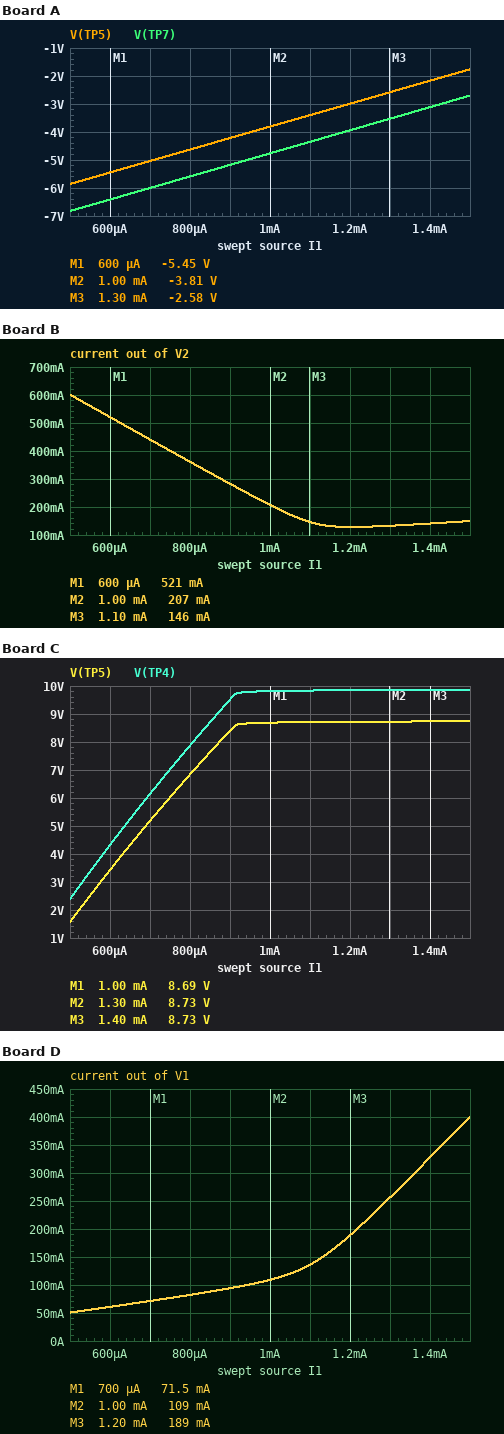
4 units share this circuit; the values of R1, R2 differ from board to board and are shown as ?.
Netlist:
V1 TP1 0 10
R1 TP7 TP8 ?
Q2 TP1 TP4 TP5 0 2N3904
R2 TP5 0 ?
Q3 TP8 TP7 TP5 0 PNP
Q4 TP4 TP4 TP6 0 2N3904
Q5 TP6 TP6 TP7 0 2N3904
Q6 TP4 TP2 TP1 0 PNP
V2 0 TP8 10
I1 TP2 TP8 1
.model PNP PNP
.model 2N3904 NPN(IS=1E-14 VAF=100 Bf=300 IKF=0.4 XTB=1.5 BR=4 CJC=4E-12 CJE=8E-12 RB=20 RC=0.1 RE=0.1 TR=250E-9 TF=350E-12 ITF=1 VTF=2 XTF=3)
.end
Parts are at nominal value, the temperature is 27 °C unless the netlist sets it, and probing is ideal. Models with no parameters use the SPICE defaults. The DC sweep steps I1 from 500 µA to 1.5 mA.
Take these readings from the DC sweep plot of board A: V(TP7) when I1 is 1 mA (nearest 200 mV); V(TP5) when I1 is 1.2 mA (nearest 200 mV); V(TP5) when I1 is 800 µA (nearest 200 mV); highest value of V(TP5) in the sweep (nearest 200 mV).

-4.8 V
-3.0 V
-4.6 V
-1.8 V
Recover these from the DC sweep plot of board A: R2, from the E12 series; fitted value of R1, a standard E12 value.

3.3 Ω
47 Ω
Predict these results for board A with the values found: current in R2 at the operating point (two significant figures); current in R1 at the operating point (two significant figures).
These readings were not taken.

2.4 A
390 mA
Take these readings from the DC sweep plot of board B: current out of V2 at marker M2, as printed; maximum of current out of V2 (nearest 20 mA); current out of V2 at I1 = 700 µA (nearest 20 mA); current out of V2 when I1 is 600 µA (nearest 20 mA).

207 mA
600 mA
440 mA
520 mA
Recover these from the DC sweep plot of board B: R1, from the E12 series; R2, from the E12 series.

82 Ω
8.2 Ω
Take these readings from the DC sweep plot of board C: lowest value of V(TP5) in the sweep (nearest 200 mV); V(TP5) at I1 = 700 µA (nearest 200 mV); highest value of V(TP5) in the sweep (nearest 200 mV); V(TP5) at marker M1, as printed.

1.6 V
5.2 V
8.8 V
8.69 V
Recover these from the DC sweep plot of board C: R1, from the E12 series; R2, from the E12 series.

220 Ω
10 Ω
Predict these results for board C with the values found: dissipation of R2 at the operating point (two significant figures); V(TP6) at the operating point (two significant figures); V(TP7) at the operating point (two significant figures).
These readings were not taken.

7.8 W
9.2 V
8.4 V
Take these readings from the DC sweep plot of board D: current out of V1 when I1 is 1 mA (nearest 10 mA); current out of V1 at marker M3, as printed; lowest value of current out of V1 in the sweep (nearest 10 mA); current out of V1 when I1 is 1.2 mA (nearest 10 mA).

110 mA
189 mA
50 mA
190 mA
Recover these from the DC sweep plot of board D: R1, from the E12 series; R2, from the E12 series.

82 Ω
12 Ω
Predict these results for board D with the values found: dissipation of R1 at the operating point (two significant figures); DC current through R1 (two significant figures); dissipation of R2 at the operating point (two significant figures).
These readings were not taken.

4.1 W
220 mA
6.6 W
